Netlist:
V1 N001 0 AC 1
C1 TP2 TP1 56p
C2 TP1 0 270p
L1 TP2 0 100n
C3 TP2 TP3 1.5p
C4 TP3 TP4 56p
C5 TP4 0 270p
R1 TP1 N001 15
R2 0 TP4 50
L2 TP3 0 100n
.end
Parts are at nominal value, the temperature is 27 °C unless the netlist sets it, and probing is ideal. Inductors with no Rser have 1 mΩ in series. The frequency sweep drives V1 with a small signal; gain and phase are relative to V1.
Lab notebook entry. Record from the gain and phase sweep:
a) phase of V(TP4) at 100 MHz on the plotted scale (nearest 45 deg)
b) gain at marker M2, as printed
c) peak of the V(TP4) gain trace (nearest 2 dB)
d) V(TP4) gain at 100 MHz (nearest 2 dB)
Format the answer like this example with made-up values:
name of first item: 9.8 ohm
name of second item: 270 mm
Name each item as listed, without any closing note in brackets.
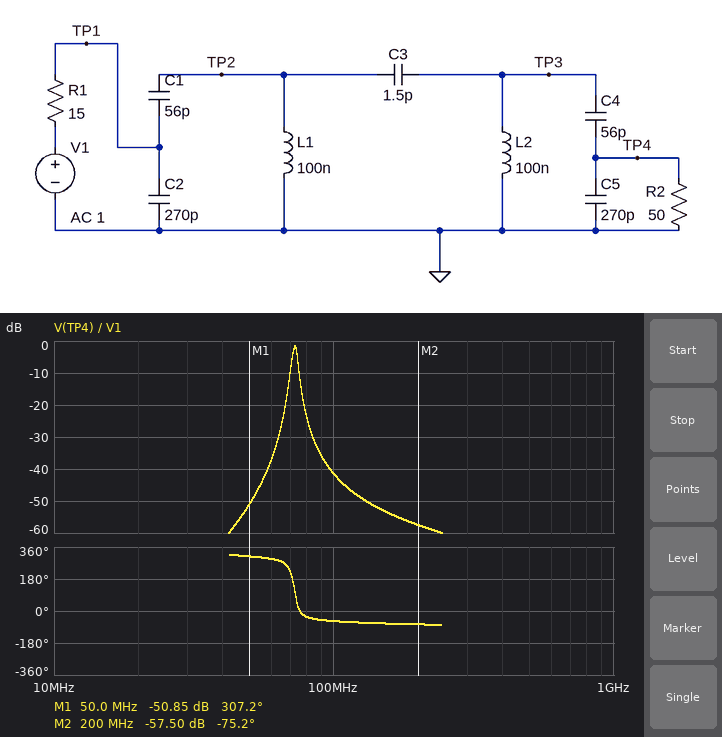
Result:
phase of V(TP4) at 100 MHz on the plotted scale: -45 deg
gain at marker M2, as printed: -57.50 dB
peak of the V(TP4) gain trace: -2 dB
V(TP4) gain at 100 MHz: -42 dB
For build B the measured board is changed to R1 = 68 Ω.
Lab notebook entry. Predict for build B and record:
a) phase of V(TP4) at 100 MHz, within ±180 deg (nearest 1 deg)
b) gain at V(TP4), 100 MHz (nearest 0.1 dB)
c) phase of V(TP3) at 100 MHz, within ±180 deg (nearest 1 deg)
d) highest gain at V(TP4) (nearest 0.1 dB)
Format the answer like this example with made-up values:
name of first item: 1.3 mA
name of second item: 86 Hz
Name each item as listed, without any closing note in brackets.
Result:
phase of V(TP4) at 100 MHz, within ±180 deg: -76 deg
gain at V(TP4), 100 MHz: -53.9 dB
phase of V(TP3) at 100 MHz, within ±180 deg: -82 deg
highest gain at V(TP4): -7.4 dB
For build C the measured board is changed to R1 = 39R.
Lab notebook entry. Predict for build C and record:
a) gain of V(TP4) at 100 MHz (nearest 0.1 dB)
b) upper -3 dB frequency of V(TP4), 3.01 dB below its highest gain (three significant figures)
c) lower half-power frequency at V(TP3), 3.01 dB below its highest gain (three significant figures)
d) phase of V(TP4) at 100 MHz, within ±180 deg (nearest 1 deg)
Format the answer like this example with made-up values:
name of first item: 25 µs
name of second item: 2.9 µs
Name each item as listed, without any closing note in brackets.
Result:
gain of V(TP4) at 100 MHz: -49.2 dB
upper -3 dB frequency of V(TP4), 3.01 dB below its highest gain: 74.2 MHz
lower half-power frequency at V(TP3), 3.01 dB below its highest gain: 71.0 MHz
phase of V(TP4) at 100 MHz, within ±180 deg: -72 deg
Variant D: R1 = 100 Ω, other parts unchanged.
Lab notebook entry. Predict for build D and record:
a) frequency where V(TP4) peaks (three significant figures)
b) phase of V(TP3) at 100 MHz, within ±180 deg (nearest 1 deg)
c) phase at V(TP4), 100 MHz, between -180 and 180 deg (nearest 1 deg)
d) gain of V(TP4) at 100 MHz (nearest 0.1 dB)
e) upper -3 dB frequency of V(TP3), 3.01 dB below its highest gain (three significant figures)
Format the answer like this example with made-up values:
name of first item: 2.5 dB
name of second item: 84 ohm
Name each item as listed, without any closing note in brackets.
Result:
frequency where V(TP4) peaks: 73.5 MHz
phase of V(TP3) at 100 MHz, within ±180 deg: -84 deg
phase at V(TP4), 100 MHz, between -180 and 180 deg: -78 deg
gain of V(TP4) at 100 MHz: -57.2 dB
upper -3 dB frequency of V(TP3), 3.01 dB below its highest gain: 74.2 MHz
